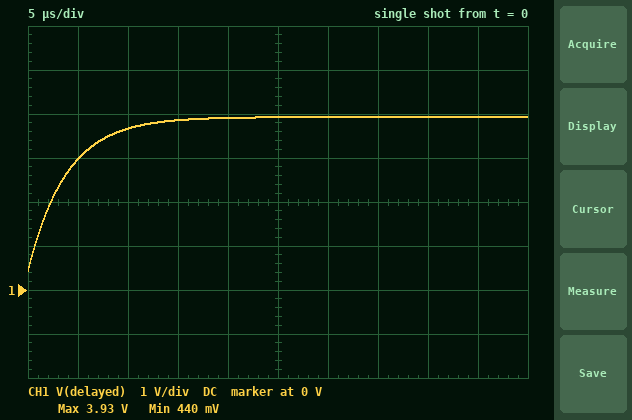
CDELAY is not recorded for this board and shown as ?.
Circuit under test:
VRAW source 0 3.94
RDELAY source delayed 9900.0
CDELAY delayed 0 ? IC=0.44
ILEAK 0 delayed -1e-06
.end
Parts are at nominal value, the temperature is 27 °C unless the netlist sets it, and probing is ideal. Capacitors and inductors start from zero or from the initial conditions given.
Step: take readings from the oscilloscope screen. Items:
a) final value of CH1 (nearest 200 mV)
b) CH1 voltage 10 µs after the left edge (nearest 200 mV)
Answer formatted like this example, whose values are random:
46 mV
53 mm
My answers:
4.0 V
3.6 V
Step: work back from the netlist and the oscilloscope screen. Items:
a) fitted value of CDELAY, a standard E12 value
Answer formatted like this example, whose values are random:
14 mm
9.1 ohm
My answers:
390 pF
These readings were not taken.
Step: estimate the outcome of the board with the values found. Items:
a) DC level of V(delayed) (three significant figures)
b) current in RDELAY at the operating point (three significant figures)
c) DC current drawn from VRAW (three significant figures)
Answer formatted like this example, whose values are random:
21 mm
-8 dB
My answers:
3.93 V
1.00 µA
1.00 µA
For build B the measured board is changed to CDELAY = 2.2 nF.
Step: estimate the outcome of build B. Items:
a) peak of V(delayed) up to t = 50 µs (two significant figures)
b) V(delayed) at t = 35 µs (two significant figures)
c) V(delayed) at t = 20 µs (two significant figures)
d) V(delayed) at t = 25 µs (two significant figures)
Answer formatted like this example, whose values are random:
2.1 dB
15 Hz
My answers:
3.6 V
3.2 V
2.5 V
2.8 V
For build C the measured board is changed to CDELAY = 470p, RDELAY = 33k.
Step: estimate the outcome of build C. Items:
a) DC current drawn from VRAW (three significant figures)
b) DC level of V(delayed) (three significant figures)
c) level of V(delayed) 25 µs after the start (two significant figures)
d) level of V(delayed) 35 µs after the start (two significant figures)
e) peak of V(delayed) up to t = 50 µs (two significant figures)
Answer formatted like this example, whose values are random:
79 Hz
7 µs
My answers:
1.00 µA
3.91 V
3.2 V
3.5 V
3.8 V
